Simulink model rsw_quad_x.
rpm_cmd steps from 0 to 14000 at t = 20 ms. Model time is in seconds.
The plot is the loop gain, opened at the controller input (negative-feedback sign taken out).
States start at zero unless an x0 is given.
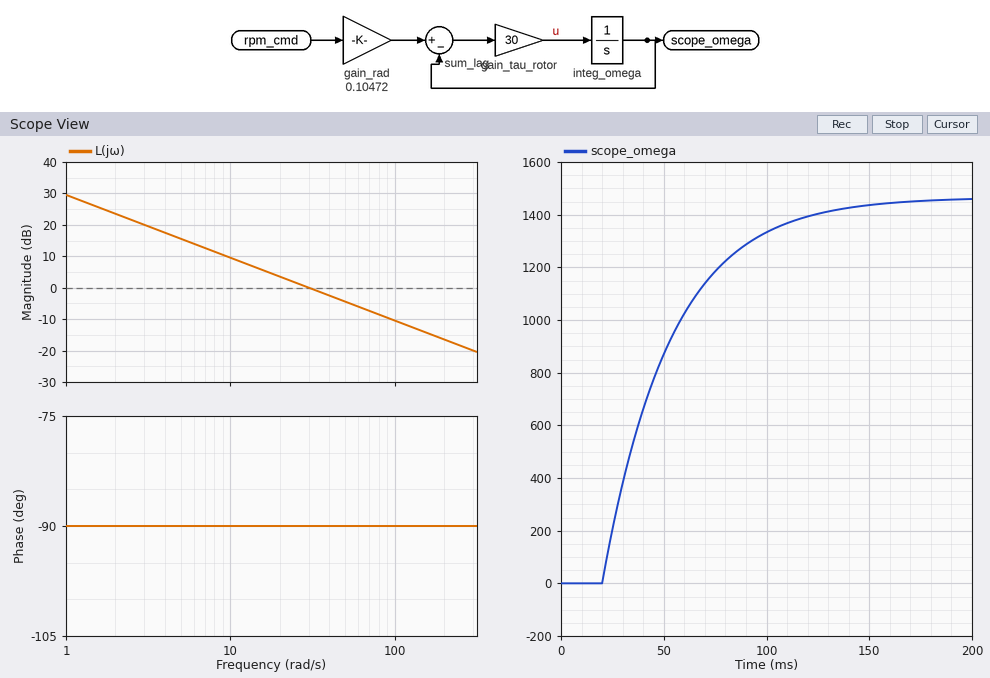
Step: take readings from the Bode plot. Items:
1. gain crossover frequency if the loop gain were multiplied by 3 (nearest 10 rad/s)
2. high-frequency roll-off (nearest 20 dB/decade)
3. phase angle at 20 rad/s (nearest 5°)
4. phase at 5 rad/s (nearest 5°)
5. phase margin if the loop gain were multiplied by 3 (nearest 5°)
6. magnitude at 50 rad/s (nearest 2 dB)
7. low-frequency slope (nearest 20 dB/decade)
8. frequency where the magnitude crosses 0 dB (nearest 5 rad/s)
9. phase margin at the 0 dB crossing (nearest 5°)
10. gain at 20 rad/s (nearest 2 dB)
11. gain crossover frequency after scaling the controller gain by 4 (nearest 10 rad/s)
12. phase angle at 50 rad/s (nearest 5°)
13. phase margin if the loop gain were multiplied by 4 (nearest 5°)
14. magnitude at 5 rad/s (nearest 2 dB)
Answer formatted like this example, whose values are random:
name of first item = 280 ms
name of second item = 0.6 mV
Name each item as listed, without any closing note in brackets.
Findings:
gain crossover frequency if the loop gain were multiplied by 3 = 90 rad/s
high-frequency roll-off = -20 dB/decade
phase angle at 20 rad/s = -90°
phase at 5 rad/s = -90°
phase margin if the loop gain were multiplied by 3 = 90°
magnitude at 50 rad/s = -4 dB
low-frequency slope = -20 dB/decade
frequency where the magnitude crosses 0 dB = 30 rad/s
phase margin at the 0 dB crossing = 90°
gain at 20 rad/s = 4 dB
gain crossover frequency after scaling the controller gain by 4 = 120 rad/s
phase angle at 50 rad/s = -90°
phase margin if the loop gain were multiplied by 4 = 90°
magnitude at 5 rad/s = 16 dB
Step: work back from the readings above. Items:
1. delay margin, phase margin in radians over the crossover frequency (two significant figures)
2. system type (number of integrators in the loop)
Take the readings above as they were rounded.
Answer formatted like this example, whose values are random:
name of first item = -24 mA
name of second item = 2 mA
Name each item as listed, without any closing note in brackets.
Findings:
delay margin, phase margin in radians over the crossover frequency = 0.052 s
system type = 1
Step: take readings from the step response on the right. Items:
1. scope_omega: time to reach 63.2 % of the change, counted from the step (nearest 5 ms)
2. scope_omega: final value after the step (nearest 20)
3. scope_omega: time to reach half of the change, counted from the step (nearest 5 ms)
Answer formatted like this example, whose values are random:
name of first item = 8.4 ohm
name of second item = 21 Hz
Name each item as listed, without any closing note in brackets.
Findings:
scope_omega: time to reach 63.2 % of the change, counted from the step = 35 ms
scope_omega: final value after the step = 1460
scope_omega: time to reach half of the change, counted from the step = 25 ms
